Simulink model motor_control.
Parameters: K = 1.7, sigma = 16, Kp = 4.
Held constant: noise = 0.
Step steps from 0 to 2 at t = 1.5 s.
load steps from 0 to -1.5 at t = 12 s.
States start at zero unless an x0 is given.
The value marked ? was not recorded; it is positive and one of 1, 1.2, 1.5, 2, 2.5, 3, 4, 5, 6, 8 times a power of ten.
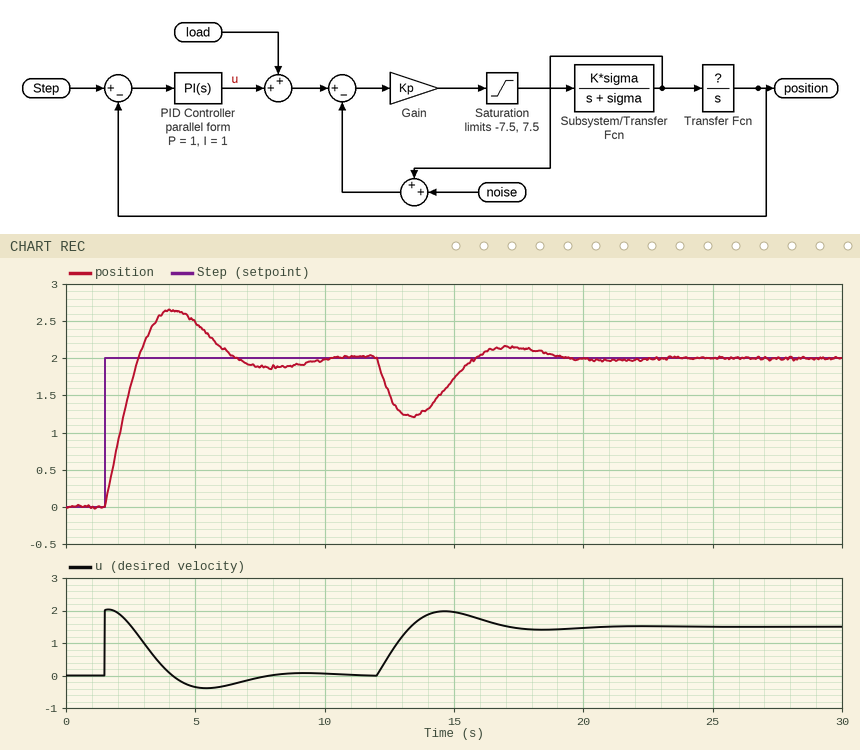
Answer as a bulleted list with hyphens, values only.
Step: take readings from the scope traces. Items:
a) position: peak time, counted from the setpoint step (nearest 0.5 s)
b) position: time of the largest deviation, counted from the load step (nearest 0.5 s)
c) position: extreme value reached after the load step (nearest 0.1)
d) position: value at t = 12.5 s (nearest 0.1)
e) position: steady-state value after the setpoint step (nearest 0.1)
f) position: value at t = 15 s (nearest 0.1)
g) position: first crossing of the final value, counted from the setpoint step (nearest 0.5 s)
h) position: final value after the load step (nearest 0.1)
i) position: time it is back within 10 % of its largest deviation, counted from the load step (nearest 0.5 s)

- 2.5 s
- 1.5 s
- 1.2
- 1.5
- 2.0
- 1.7
- 1.5 s
- 2.0
- 6.5 s
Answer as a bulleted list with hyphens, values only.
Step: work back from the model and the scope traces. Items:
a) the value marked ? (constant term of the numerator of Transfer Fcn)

- 1
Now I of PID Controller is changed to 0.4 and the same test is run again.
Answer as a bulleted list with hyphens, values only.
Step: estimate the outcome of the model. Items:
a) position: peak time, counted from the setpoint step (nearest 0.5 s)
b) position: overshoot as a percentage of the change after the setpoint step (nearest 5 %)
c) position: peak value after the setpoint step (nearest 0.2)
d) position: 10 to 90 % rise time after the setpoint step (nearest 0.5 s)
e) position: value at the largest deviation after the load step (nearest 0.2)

- 3.5 s
- 20 %
- 2.4
- 1.5 s
- 1.0
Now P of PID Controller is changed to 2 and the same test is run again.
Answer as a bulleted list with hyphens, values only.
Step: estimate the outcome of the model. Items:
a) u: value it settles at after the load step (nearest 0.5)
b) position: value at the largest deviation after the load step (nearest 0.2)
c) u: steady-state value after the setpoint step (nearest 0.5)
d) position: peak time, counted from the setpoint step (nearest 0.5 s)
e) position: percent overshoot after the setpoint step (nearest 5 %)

- 1.5
- 1.4
- 0.0
- 2.0 s
- 15 %
